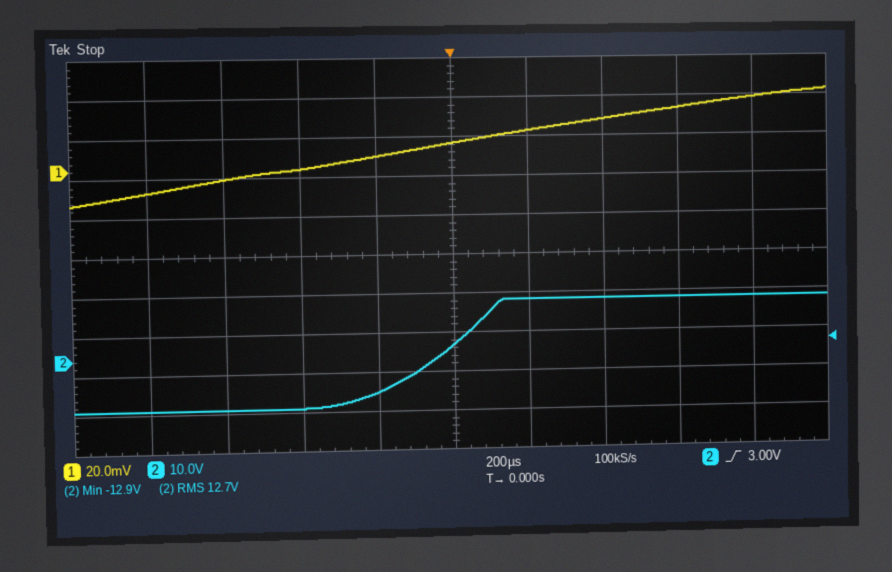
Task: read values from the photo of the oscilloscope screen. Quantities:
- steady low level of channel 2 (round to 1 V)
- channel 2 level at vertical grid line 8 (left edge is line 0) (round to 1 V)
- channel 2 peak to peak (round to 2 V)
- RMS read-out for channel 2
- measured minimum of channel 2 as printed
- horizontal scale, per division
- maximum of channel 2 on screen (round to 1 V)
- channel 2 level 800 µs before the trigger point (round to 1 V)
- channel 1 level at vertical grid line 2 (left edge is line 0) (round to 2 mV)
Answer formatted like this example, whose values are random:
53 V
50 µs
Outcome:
-13 V
14 V
28 V
12.7 V
-12.9 V
200 µs
14 V
-13 V
-4 mV
